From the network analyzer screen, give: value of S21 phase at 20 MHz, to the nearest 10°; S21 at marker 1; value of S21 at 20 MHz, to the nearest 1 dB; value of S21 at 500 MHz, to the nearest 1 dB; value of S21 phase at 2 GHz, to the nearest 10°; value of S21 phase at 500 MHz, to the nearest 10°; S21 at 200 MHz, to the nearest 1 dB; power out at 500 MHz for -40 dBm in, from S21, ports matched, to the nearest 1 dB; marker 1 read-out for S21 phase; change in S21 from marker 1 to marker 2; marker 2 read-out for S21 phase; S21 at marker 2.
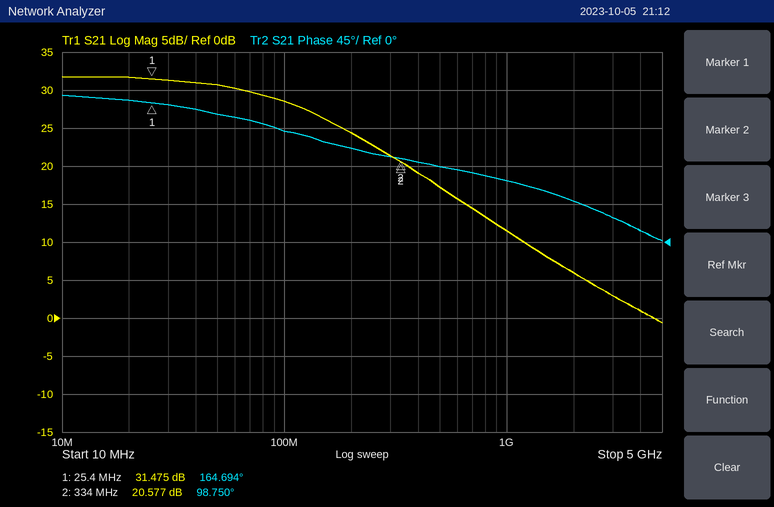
170°
31.475 dB
32 dB
17 dB
50°
90°
24 dB
-23 dBm
164.694°
-10.898 dB
98.750°
20.577 dB
